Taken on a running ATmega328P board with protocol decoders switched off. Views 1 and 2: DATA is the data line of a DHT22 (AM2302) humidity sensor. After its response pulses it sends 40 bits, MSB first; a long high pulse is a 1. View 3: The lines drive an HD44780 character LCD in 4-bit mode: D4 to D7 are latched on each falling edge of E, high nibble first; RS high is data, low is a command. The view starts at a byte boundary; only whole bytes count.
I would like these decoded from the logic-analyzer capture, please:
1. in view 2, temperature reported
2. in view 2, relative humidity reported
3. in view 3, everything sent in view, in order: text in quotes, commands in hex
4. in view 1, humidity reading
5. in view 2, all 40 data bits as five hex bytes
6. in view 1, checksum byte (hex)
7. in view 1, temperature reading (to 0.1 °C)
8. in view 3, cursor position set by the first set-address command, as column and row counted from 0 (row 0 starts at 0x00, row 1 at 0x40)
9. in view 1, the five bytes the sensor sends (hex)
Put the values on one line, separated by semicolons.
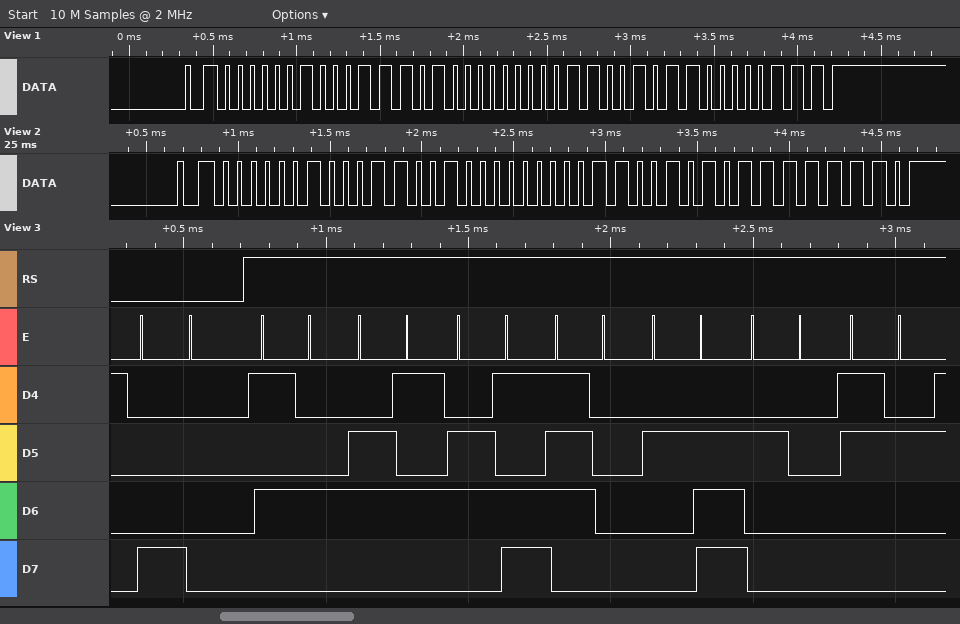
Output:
20.2 °C; 56.2 %; 0x80 "Temp. 2"; 57.0 %; 02 32 00 CA FE; 0x07; 20.3 °C; column 0, row 0; 02 3A 00 CB 07
